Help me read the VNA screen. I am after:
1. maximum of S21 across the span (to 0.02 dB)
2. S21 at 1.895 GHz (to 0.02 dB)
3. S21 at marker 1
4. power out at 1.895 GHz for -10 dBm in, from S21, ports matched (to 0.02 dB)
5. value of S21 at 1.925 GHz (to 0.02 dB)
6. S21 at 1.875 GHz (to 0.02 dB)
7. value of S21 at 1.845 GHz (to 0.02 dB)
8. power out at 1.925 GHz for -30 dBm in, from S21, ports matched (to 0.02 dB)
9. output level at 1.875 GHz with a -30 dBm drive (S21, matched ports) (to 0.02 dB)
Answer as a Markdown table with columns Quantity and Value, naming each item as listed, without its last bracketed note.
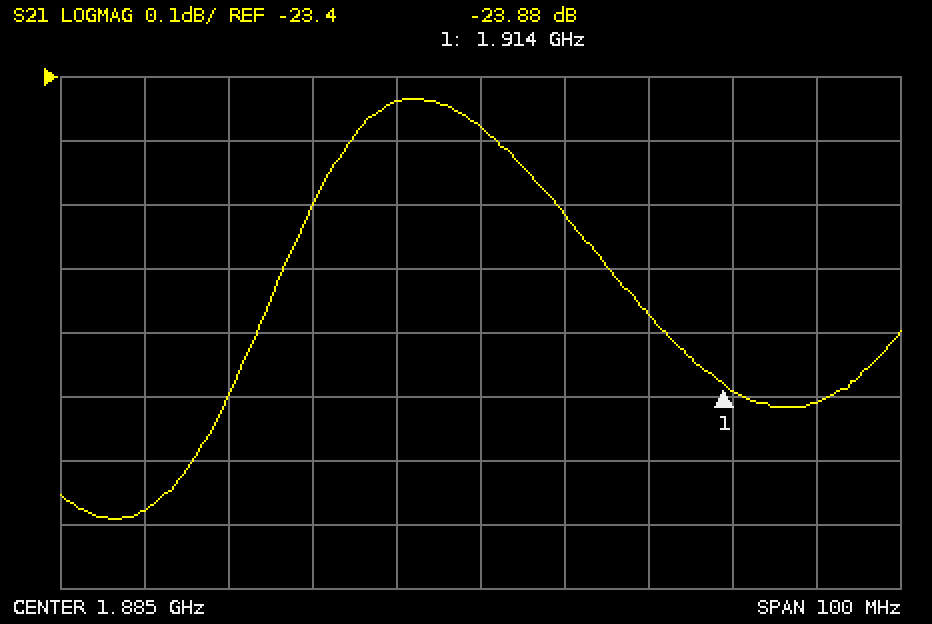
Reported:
| Quantity | Value |
|---|---|
| maximum of S21 across the span | -23.44 dB |
| S21 at 1.895 GHz | -23.62 dB |
| S21 at marker 1 | -23.88 dB |
| power out at 1.895 GHz for -10 dBm in, from S21, ports matched | -33.62 dBm |
| value of S21 at 1.925 GHz | -23.90 dB |
| S21 at 1.875 GHz | -23.44 dB |
| value of S21 at 1.845 GHz | -24.08 dB |
| power out at 1.925 GHz for -30 dBm in, from S21, ports matched | -53.90 dBm |
| output level at 1.875 GHz with a -30 dBm drive (S21, matched ports) | -53.44 dBm |
